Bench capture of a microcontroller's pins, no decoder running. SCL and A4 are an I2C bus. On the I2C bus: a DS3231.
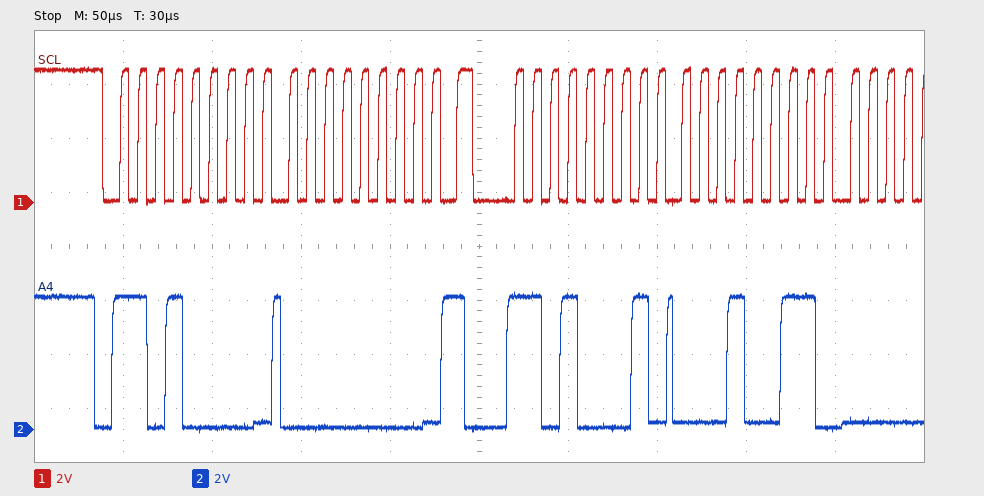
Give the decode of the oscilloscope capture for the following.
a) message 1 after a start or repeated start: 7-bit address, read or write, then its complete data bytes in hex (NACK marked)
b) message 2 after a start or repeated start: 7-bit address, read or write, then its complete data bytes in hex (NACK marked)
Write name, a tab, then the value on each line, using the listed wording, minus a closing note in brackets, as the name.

message 1 after a start or repeated start: 7-bit address, read or write, then its complete data bytes in hex	0x68 write: 00
message 2 after a start or repeated start: 7-bit address, read or write, then its complete data bytes in hex	0x68 read: 13
